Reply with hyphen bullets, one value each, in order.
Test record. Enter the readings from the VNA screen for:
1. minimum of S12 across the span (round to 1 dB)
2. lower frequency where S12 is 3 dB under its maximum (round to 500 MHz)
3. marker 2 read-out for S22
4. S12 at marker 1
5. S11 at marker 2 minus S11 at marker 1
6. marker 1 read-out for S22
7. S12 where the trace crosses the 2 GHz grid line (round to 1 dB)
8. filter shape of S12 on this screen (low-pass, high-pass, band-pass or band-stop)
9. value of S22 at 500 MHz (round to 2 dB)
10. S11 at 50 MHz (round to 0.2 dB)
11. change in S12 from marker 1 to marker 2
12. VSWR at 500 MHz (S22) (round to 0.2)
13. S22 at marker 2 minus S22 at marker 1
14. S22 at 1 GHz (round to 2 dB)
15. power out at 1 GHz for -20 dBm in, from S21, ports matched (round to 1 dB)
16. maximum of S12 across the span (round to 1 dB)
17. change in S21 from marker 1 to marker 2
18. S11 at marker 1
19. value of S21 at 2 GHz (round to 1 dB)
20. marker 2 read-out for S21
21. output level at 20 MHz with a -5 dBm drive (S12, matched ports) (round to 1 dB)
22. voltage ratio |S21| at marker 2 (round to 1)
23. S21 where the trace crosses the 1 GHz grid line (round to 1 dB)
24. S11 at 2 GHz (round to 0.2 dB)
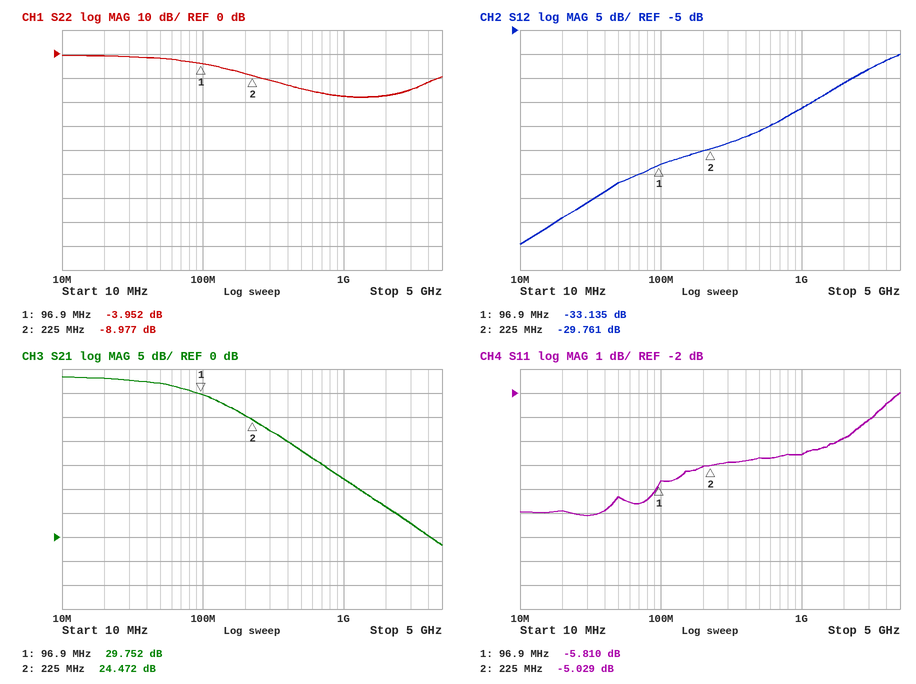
- -50 dB
- 3.0 GHz
- -8.977 dB
- -33.135 dB
- 0.781 dB
- -3.952 dB
- -16 dB
- high-pass
- -14 dB
- -6.4 dB
- 3.374 dB
- 1.4
- -5.025 dB
- -18 dB
- -8 dBm
- -10 dB
- -5.280 dB
- -5.810 dB
- 6 dB
- 24.472 dB
- -49 dBm
- 17
- 12 dB
- -3.8 dB
